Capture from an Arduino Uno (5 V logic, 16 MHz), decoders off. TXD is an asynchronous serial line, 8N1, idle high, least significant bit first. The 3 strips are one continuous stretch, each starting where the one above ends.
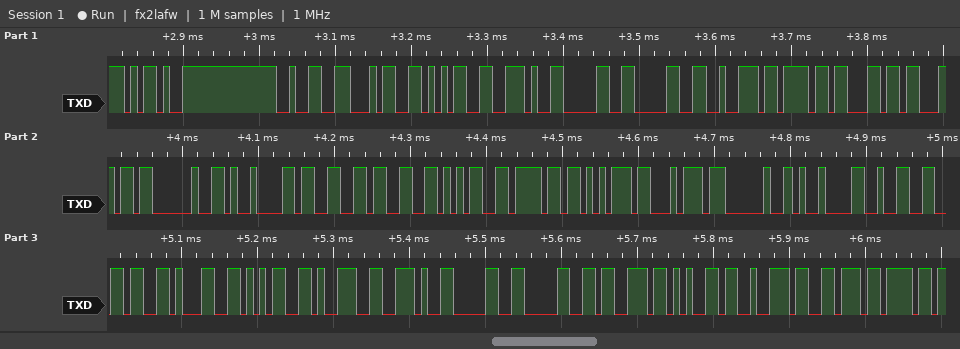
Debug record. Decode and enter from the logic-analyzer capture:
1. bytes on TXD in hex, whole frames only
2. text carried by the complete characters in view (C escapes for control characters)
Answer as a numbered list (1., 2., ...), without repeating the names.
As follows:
1. 0x2D 0x32 0x34 0x35 0x2E 0x30 0x30 0x72 0x6F 0x6C 0x6C 0x20 0x09 0x33 0x33 0x35 0x6F 0x75 0x74 0x20 0x09 0x32 0x36 0x31 0x35 0x39 0x2E 0x30 0x30 0x73 0x65 0x72 0x76 0x6F
2. "-245.00roll \t335out \t26159.00servo"
